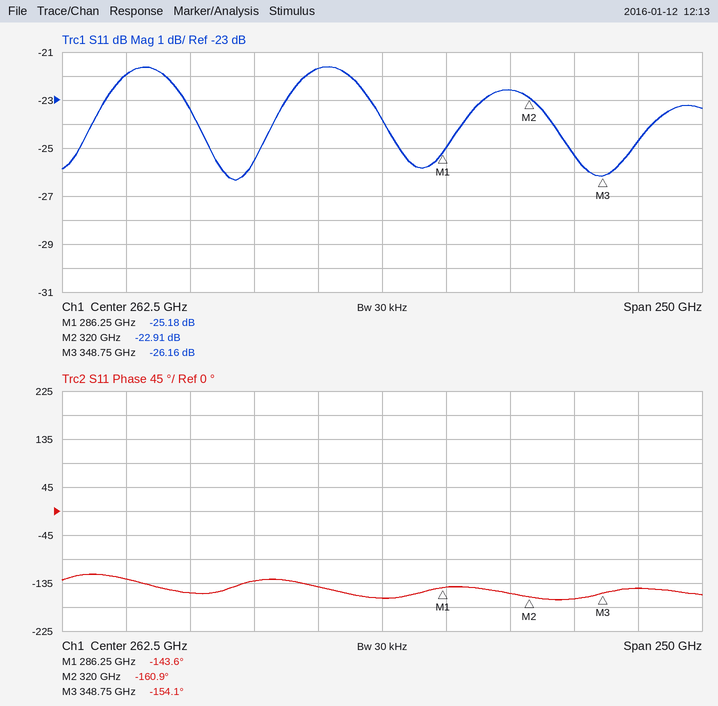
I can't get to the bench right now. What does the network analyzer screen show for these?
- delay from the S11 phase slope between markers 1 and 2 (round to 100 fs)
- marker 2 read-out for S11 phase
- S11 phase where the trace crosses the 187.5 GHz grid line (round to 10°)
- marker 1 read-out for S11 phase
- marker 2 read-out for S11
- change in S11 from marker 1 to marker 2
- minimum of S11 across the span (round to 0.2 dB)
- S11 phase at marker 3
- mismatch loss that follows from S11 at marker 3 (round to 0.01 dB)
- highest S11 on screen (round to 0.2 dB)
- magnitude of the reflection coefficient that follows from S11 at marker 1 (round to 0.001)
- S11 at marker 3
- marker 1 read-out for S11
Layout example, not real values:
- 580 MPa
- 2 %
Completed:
- 1.4 ps
- -160.9°
- -150°
- -143.6°
- -22.91 dB
- 2.27 dB
- -26.4 dB
- -154.1°
- 0.01 dB
- -21.6 dB
- 0.055
- -26.16 dB
- -25.18 dB
